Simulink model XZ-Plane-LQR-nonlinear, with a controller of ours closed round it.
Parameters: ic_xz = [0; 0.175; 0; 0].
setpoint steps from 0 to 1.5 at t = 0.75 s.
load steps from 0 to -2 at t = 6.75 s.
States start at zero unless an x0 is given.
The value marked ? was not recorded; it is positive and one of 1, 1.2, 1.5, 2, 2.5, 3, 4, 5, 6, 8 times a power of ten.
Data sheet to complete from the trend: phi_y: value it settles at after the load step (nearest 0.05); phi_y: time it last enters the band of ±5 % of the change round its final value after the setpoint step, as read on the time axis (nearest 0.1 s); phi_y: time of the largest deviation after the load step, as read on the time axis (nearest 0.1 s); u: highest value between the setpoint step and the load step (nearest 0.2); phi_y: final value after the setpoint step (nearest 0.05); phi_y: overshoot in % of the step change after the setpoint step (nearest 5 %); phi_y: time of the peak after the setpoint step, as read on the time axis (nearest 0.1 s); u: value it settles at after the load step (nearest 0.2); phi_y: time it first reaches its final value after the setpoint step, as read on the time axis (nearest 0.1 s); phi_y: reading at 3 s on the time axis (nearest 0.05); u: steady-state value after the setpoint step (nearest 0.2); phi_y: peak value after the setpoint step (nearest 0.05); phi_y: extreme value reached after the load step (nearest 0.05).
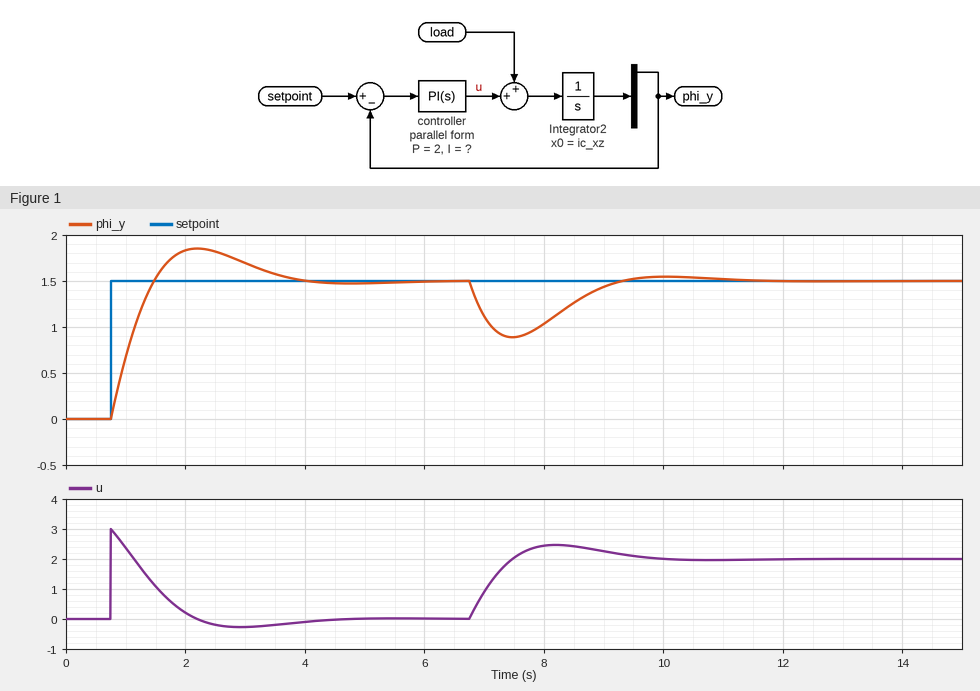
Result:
1.50
3.5 s
7.5 s
3.0
1.50
25 %
2.2 s
2.0
1.5 s
1.70
0.0
1.85
0.90
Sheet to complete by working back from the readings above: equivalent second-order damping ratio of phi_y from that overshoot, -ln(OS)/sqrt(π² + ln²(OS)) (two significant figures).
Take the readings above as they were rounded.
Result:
0.40
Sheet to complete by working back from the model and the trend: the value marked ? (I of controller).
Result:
2.5
